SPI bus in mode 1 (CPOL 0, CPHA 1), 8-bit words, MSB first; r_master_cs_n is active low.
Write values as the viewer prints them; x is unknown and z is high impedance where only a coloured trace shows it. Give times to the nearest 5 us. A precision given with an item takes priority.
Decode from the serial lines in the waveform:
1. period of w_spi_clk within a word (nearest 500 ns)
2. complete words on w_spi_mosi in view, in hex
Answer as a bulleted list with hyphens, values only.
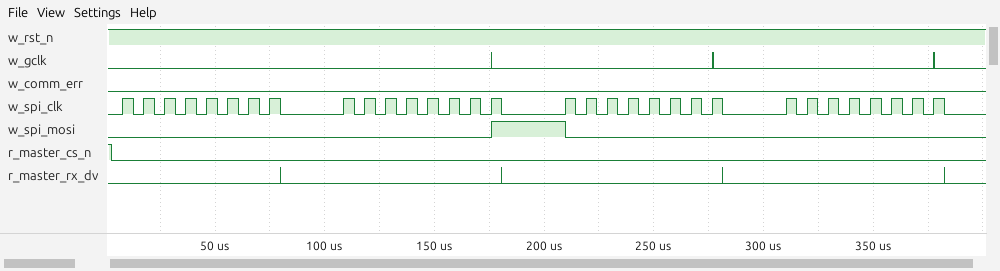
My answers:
- 9500 ns
- 00, 01, 00, 00
